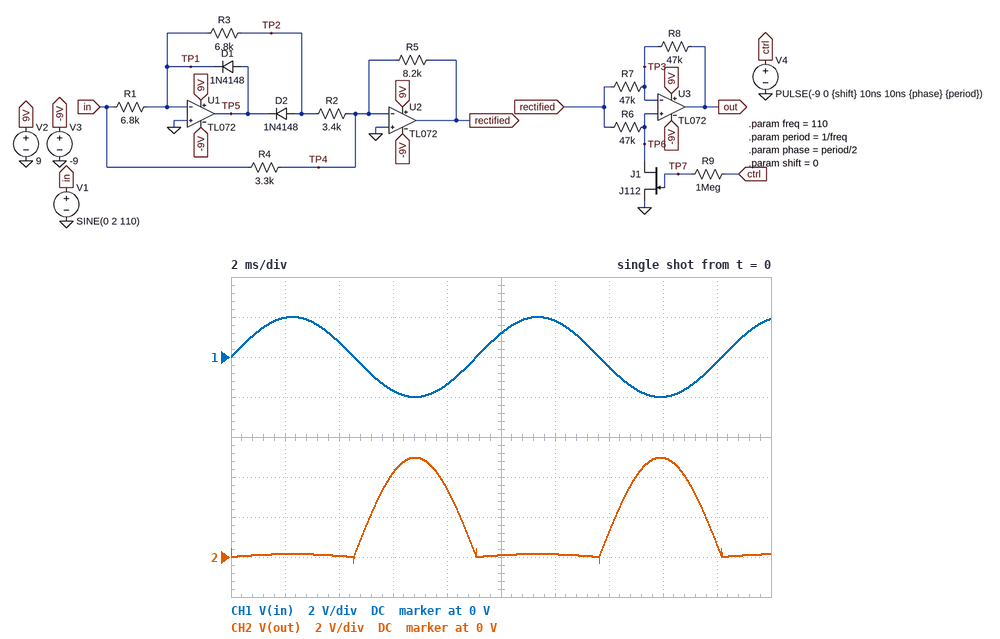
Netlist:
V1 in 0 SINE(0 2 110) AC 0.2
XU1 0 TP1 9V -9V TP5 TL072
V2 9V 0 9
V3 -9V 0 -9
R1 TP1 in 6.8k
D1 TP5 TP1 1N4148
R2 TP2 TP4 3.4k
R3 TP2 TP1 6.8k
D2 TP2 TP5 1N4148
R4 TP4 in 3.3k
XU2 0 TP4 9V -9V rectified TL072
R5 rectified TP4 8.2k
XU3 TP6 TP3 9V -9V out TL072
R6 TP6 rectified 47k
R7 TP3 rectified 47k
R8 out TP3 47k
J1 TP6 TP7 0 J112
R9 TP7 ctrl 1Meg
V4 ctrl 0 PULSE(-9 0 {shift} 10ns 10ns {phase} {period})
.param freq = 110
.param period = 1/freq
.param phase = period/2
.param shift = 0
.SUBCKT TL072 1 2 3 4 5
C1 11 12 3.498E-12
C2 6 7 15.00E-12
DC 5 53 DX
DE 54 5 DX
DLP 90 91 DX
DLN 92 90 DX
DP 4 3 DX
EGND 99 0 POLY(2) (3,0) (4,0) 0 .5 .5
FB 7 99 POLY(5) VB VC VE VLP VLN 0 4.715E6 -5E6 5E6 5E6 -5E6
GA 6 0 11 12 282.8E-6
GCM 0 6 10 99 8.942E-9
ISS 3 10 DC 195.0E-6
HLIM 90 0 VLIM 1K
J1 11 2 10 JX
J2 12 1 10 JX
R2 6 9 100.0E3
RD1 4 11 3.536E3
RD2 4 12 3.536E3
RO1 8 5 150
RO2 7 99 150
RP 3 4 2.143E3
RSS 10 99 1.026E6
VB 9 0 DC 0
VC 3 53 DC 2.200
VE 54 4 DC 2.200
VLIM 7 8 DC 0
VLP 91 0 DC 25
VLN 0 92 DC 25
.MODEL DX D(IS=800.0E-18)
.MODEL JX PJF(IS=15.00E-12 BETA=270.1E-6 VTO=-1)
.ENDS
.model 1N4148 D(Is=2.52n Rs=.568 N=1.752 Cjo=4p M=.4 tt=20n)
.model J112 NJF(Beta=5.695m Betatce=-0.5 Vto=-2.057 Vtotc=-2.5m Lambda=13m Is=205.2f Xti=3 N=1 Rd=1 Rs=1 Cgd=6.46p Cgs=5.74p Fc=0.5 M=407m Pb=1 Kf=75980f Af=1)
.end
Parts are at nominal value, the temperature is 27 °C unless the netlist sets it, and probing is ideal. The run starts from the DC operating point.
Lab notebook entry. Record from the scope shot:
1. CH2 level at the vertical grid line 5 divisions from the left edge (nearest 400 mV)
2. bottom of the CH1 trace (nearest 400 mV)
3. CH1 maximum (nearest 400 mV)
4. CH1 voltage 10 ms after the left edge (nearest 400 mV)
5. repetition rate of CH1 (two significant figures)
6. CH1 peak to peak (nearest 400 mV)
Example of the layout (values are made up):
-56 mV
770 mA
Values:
0 V
-2.0 V
2.0 V
1.2 V
110 Hz
4.0 V
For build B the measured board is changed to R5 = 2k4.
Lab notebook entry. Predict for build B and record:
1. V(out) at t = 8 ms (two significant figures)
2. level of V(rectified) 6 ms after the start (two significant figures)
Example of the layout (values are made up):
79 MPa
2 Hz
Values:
1.0 V
1.2 V
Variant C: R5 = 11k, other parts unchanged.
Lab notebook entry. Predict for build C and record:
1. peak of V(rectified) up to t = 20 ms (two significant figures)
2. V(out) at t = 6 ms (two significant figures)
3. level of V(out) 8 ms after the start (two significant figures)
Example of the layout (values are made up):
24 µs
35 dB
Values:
6.7 V
5.6 V
4.6 V
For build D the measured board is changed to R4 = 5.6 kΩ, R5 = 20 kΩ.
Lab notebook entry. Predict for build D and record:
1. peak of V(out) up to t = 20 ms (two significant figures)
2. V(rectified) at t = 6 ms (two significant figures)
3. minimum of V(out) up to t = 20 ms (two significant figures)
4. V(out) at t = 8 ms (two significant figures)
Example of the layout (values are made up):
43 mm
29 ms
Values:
7.1 V
6.0 V
-4.6 V
4.9 V
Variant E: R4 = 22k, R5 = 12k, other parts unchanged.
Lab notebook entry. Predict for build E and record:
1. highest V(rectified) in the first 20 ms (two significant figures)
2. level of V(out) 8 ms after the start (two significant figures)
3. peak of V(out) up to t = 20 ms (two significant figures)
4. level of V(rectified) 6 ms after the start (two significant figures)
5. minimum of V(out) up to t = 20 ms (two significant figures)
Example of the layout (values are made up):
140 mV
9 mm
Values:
6.0 V
750 mV
1.1 V
920 mV
-6.0 V
